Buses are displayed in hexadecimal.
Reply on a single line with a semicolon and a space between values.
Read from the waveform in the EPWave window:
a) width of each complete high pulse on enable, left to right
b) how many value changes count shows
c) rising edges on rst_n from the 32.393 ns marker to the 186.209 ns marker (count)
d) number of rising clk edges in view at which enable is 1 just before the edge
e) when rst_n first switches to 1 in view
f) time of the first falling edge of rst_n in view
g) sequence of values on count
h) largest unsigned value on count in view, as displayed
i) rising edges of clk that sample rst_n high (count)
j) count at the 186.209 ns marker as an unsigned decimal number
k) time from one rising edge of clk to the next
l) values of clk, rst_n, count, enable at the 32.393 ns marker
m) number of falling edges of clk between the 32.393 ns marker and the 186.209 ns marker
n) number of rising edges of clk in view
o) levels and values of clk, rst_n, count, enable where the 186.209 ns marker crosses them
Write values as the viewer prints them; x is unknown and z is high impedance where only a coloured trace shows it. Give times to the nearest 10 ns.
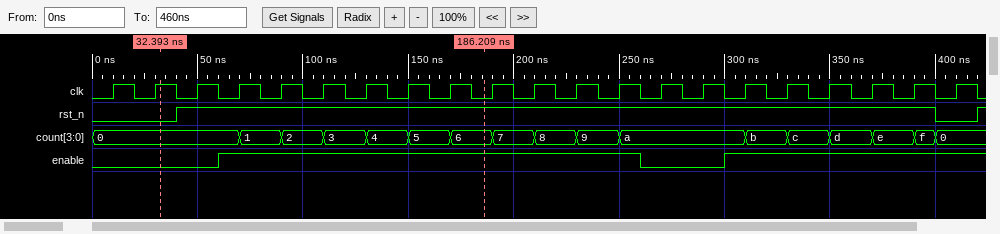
200 ns; 16; 1; 16; 40 ns; 400 ns; 0, 1, 2, 3, 4, 5, 6, 7, 8, 9, a, b, c, d, e, f, 0; f; 18; 6; 20 ns; clk=1, rst_n=0, count=0, enable=0; 8; 21; clk=0, rst_n=1, count=6, enable=1
